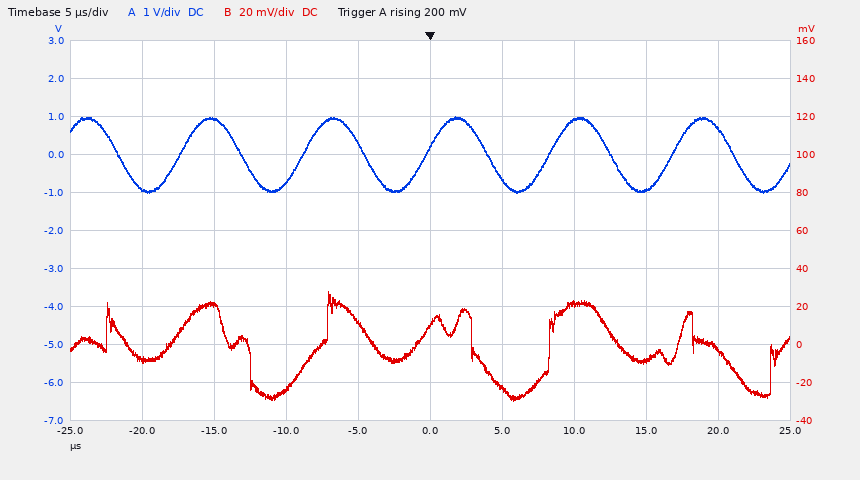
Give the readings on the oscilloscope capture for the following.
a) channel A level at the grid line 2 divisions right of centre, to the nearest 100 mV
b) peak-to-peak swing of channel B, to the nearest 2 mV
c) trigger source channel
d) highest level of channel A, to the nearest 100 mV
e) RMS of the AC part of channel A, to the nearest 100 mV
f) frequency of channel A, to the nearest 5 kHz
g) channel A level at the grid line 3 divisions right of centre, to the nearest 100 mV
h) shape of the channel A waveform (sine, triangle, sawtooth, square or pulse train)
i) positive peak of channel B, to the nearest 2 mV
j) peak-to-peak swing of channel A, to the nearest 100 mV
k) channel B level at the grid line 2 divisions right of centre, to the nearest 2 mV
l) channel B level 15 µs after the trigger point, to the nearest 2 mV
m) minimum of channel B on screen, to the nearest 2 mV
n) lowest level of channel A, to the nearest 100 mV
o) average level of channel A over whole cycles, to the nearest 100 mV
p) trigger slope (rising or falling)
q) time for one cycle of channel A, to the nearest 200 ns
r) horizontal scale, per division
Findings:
900 mV
58 mV
channel A
1.0 V
700 mV
115 kHz
-900 mV
sine
28 mV
2.0 V
22 mV
-8 mV
-30 mV
-1.0 V
0.0 V
rising
8.6 µs
5 µs
